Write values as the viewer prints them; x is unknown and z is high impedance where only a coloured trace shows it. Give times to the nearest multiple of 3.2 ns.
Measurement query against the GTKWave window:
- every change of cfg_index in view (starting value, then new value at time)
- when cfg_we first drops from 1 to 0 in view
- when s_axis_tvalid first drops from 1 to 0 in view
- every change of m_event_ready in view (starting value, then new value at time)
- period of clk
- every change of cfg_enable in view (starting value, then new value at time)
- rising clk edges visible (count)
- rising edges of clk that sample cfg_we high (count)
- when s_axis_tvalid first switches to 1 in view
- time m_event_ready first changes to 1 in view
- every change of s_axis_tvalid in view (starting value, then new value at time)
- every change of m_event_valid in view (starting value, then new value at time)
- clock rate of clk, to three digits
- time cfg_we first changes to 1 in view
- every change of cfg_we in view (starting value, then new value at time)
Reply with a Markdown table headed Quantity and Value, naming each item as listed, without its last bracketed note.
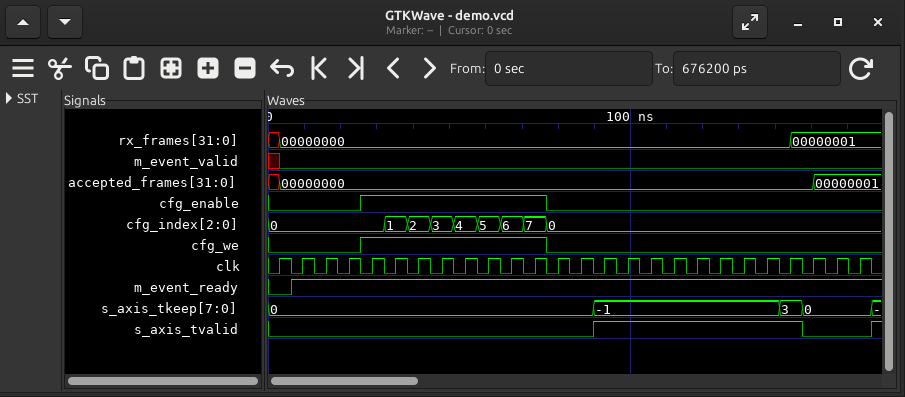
| Quantity | Value |
|---|---|
| every change of cfg_index in view | 0, 1 at 32 ns, 2 at 38.4 ns, 3 at 44.8 ns, 4 at 51.2 ns, 5 at 57.6 ns, 6 at 64 ns, 7 at 70.4 ns, 0 at 76.8 ns |
| when cfg_we first drops from 1 to 0 in view | 76.8 ns |
| when s_axis_tvalid first drops from 1 to 0 in view | 147.2 ns |
| every change of m_event_ready in view | 0, 1 at 6.4 ns |
| period of clk | 6.4 ns |
| every change of cfg_enable in view | 0, 1 at 25.6 ns, 0 at 76.8 ns |
| rising clk edges visible | 26 |
| rising edges of clk that sample cfg_we high | 8 |
| when s_axis_tvalid first switches to 1 in view | 89.6 ns |
| time m_event_ready first changes to 1 in view | 6.4 ns |
| every change of s_axis_tvalid in view | 0, 1 at 89.6 ns, 0 at 147.2 ns, 1 at 166.4 ns |
| every change of m_event_valid in view | x, 0 at 3.2 ns |
| clock rate of clk, to three digits | 156 MHz |
| time cfg_we first changes to 1 in view | 25.6 ns |
| every change of cfg_we in view | 0, 1 at 25.6 ns, 0 at 76.8 ns |
